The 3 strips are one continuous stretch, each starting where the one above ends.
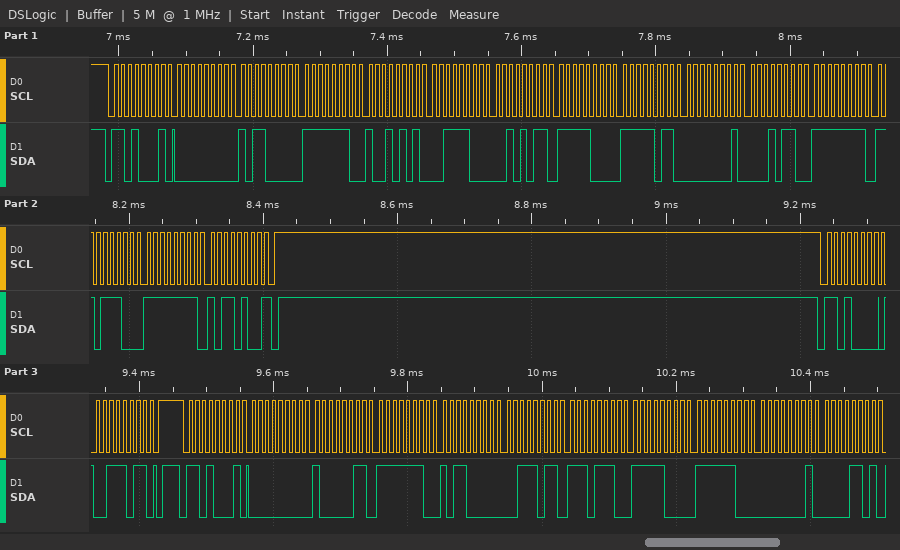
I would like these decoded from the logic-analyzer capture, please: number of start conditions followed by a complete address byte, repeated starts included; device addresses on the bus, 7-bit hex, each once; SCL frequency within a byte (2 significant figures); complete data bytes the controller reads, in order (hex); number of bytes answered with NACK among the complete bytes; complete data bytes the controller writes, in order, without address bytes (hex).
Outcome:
3
0x68
100 kHz
00 B0 FE 95 3C 2B F8 FB 01 16 FF DC FF B4 00 83 FE B0 3B EE F8 FC 01 0D
1
3B
